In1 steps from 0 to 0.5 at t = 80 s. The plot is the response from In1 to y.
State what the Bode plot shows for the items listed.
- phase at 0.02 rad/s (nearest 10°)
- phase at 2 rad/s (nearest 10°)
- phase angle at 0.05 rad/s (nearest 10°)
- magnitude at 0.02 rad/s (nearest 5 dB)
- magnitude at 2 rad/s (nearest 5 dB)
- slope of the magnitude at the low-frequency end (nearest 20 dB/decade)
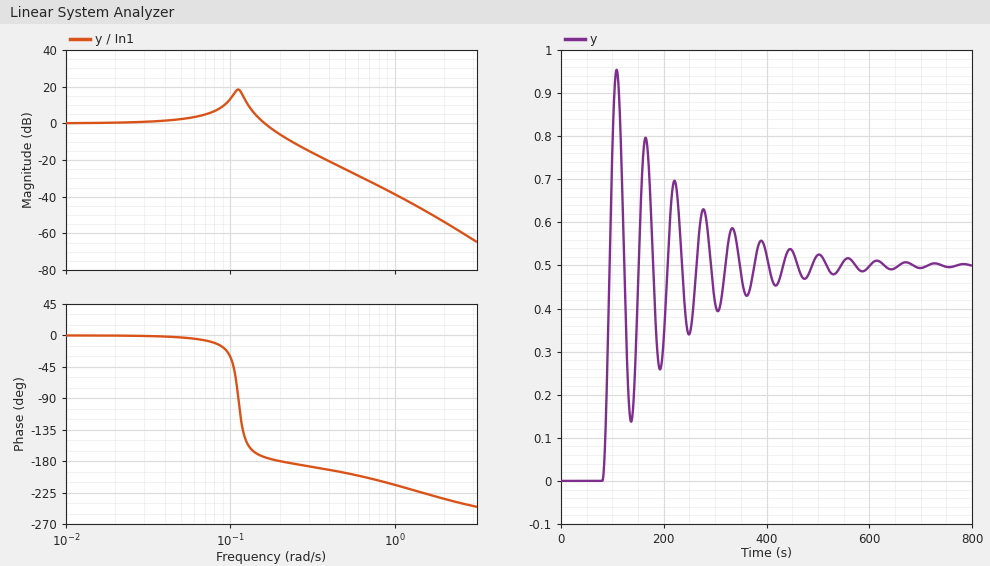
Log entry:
0°
-230°
0°
0 dB
-55 dB
0 dB/decade
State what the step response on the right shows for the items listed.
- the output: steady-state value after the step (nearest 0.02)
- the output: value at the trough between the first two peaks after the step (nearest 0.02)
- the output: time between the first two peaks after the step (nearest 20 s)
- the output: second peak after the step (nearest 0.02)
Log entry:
0.50
0.14
60 s
0.80
